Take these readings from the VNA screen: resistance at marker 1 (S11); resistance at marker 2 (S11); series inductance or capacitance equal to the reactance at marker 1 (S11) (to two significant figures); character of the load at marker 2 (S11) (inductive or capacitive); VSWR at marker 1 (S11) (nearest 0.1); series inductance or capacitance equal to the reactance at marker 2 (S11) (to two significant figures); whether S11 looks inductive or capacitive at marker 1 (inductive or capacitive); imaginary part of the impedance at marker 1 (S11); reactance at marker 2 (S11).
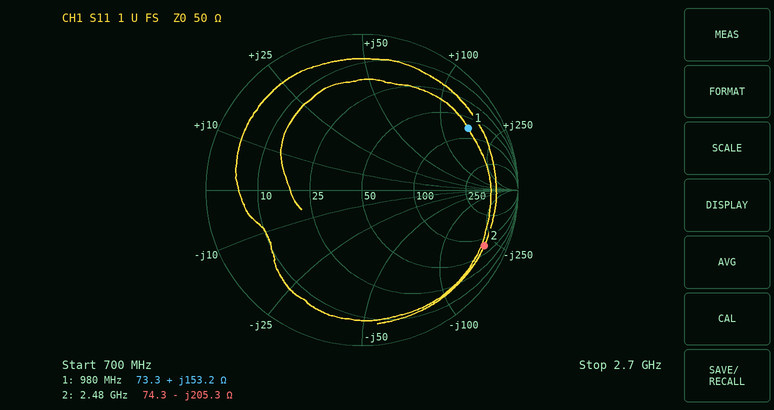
73.3 Ω
74.3 Ω
25 nH
capacitive
8.4
310 fF
inductive
+153.2 Ω
-205.3 Ω
